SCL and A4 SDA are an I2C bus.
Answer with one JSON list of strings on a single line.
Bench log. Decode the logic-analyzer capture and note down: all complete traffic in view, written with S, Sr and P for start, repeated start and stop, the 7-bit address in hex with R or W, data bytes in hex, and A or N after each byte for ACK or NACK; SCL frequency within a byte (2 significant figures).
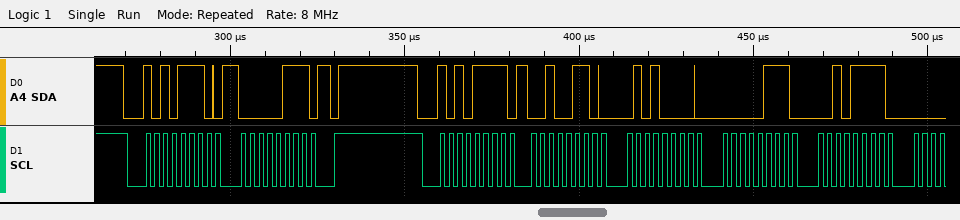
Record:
["S 57W A 07 A P S 57R A 26 A 50 A 07 A 2F A", "400 kHz"]
